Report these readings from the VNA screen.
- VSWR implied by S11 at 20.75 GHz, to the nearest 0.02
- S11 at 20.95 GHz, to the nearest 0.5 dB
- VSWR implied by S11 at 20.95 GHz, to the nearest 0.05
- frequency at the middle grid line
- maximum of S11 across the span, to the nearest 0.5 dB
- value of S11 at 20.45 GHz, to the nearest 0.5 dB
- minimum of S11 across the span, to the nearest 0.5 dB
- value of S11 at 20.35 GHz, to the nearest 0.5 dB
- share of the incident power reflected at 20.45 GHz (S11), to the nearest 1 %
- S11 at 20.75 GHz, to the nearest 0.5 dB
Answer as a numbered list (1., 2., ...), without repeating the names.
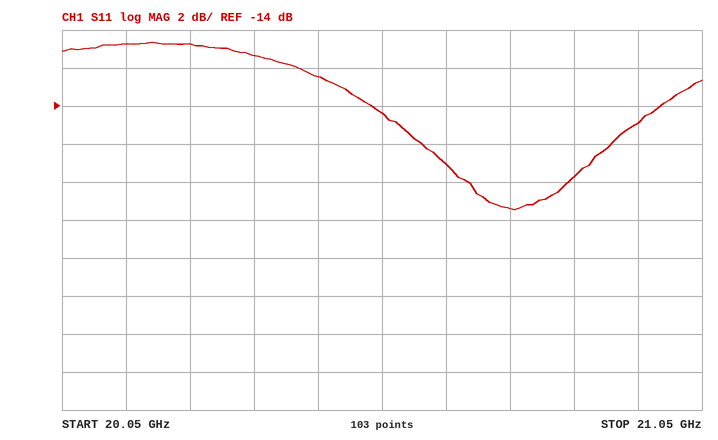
1. 1.24
2. -15.0 dB
3. 1.45
4. 20.55 GHz
5. -10.5 dB
6. -12.5 dB
7. -19.5 dB
8. -11.5 dB
9. 6 %
10. -19.5 dB
